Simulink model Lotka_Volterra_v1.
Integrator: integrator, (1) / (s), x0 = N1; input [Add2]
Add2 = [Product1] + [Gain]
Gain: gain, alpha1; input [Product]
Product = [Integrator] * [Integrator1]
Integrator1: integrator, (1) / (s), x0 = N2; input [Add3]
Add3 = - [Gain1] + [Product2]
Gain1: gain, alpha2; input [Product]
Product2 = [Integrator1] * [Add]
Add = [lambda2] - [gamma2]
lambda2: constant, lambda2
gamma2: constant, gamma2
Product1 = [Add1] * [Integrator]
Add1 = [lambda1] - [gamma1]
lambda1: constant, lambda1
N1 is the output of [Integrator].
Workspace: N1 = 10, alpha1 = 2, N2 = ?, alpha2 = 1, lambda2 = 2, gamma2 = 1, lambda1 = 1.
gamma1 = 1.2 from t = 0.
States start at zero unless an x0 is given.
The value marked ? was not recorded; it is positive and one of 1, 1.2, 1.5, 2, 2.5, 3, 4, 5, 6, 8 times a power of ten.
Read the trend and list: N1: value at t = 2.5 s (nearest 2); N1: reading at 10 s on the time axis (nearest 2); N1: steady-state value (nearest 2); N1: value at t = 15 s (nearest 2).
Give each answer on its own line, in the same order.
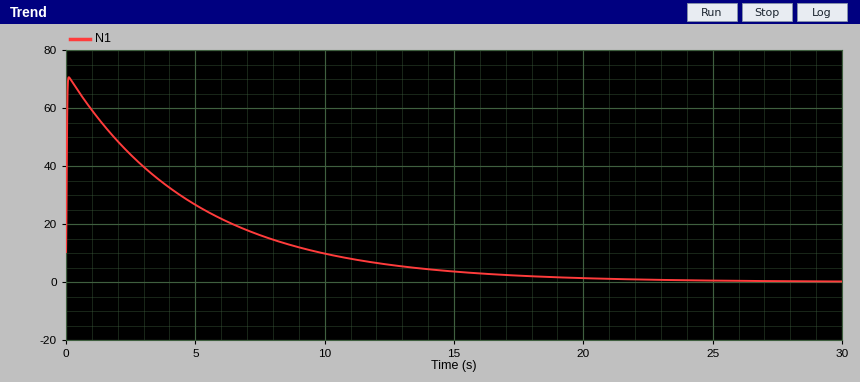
44
10
0
4
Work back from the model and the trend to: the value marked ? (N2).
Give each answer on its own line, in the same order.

30
